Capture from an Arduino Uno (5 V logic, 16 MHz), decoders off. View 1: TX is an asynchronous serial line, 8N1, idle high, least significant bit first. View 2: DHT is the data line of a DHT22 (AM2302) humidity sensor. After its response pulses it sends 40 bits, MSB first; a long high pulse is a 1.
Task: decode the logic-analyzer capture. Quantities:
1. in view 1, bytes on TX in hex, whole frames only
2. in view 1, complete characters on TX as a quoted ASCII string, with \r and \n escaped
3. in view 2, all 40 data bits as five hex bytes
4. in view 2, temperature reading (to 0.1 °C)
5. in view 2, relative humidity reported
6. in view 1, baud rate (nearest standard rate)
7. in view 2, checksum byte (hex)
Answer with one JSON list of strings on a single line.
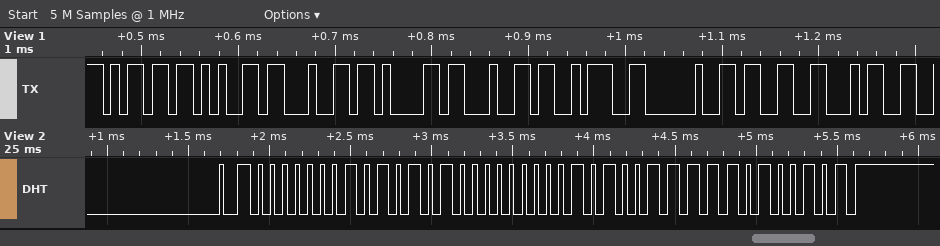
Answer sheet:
["0x6D 0x65 0x64 0x61 0x64 0x3A 0x20 0x33 0x34", "\"medad: 34\"", "01 54 01 4F A5", "33.5 °C", "34.0 %", "115200 baud", "0xA5"]
